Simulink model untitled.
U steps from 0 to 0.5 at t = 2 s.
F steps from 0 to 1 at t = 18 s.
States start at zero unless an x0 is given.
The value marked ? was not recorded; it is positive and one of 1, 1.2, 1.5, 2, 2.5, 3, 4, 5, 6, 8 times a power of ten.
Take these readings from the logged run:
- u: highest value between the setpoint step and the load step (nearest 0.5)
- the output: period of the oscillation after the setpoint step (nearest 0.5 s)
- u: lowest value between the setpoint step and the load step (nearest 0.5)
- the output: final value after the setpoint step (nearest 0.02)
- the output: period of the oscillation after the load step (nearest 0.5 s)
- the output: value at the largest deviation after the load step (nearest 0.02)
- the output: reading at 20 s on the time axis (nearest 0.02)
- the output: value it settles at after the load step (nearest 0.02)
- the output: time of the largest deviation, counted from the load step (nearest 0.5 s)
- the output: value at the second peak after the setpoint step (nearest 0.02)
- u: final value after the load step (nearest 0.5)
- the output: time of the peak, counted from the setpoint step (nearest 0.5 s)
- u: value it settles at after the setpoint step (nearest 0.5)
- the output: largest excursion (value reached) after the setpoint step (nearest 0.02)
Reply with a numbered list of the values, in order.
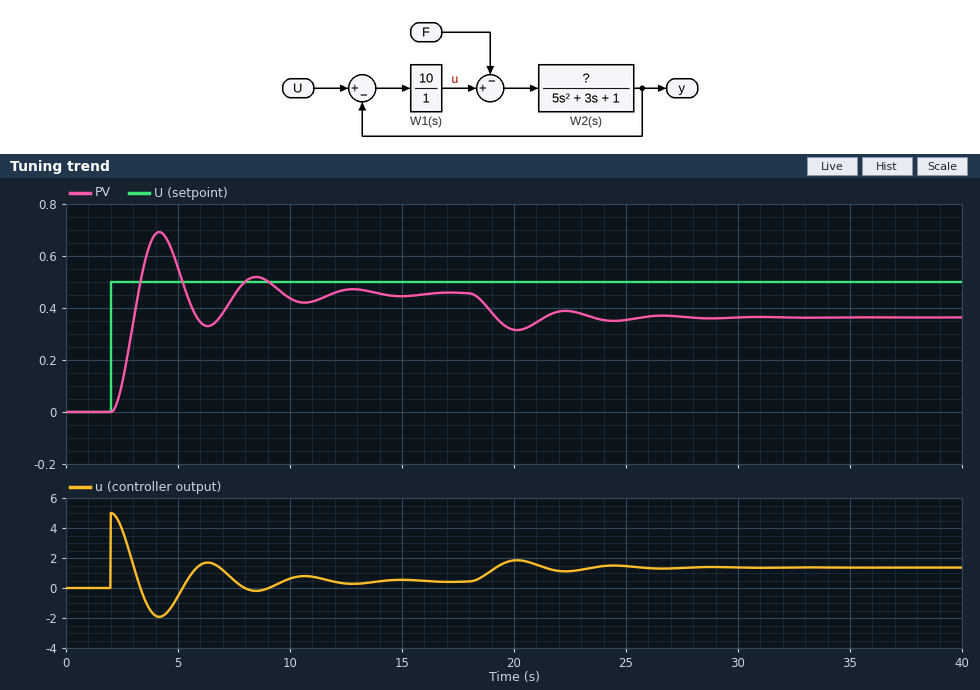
1. 5.0
2. 4.5 s
3. -2.0
4. 0.46
5. 4.5 s
6. 0.32
7. 0.32
8. 0.36
9. 2.0 s
10. 0.52
11. 1.5
12. 2.0 s
13. 0.5
14. 0.70
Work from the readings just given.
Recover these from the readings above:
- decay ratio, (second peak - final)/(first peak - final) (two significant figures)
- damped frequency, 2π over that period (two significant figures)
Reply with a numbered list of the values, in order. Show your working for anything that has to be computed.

1. (0.52 - 0.46) / (0.7 - 0.46) = 0.25
2. 2π / 4.5 = 1.4 rad/s
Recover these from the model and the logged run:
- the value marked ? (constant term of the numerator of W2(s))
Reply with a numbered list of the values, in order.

1. 1
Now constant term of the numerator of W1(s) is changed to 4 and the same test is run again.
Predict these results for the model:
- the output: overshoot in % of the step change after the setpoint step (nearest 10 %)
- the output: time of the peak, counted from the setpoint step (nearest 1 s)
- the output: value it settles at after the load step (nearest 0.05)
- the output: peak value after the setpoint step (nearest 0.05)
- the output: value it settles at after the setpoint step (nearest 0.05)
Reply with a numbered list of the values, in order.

1. 40 %
2. 3 s
3. 0.20
4. 0.55
5. 0.40
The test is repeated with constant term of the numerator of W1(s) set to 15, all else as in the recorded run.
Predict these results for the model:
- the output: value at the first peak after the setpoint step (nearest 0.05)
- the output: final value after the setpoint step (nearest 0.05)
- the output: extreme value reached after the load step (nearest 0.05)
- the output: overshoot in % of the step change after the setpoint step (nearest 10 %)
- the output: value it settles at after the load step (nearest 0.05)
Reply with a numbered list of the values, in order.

1. 0.75
2. 0.45
3. 0.35
4. 60 %
5. 0.40
